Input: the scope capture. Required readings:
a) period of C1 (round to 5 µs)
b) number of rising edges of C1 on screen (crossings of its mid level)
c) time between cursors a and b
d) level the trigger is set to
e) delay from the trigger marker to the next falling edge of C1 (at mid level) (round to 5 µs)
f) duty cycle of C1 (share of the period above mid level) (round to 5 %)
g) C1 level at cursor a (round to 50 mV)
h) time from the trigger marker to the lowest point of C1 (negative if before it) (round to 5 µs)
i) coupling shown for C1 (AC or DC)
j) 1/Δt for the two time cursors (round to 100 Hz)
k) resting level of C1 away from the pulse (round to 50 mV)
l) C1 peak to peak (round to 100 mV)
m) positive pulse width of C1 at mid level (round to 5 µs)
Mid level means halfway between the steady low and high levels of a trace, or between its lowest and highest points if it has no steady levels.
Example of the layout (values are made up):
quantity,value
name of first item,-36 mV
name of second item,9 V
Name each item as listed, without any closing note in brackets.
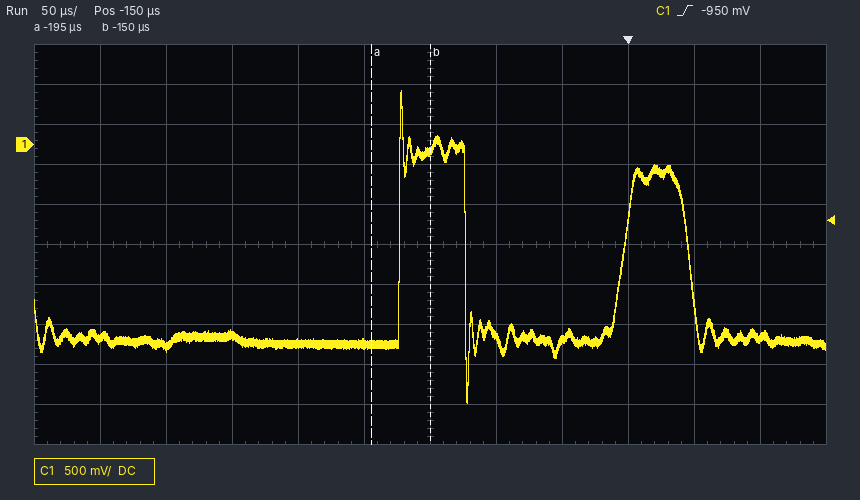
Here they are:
quantity,value
period of C1,170 µs
number of rising edges of C1 on screen,2
time between cursors a and b,45 µs
level the trigger is set to,-950 mV
delay from the trigger marker to the next falling edge of C1 (at mid level),45 µs
duty cycle of C1 (share of the period above mid level),30 %
C1 level at cursor a,-2.50 V
time from the trigger marker to the lowest point of C1 (negative if before it),-120 µs
coupling shown for C1,DC
1/Δt for the two time cursors,22.2 kHz
resting level of C1 away from the pulse,-2.45 V
C1 peak to peak,3.90 V
positive pulse width of C1 at mid level,50 µs
